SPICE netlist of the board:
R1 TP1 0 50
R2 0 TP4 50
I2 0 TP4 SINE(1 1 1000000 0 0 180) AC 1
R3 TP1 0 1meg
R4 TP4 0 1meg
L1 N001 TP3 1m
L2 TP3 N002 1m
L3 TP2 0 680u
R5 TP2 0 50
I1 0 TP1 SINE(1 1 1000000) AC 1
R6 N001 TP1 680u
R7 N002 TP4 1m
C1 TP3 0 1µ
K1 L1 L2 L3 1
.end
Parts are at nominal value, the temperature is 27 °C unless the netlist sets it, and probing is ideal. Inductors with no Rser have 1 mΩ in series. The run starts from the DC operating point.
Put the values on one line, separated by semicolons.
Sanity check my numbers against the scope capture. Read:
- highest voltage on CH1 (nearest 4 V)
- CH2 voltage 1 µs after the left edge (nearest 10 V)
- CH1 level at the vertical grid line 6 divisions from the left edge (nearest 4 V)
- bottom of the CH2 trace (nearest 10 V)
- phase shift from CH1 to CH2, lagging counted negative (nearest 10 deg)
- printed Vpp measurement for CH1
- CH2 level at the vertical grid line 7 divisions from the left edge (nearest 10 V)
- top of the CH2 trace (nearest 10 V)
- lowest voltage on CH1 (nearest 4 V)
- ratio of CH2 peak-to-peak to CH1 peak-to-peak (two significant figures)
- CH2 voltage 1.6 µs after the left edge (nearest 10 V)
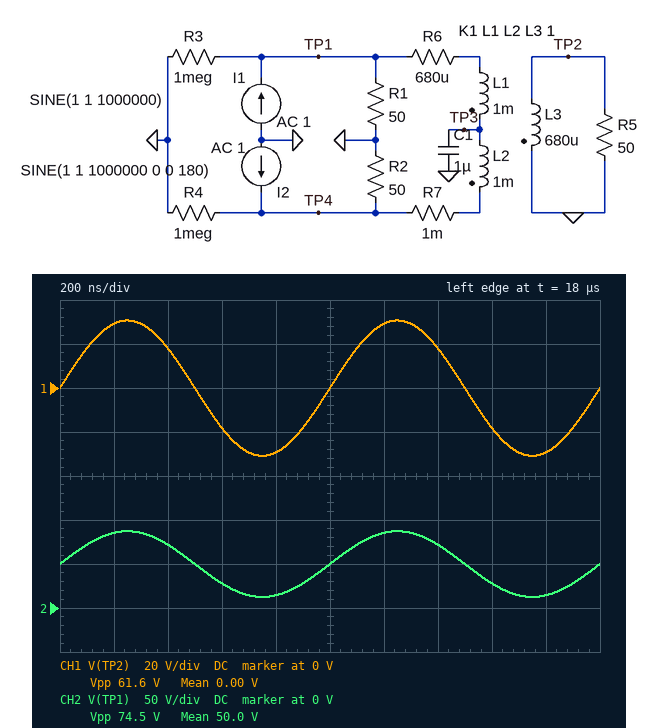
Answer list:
32 V; 50 V; 28 V; 10 V; 0 deg; 61.6 V; 70 V; 90 V; -32 V; 1.2; 30 V
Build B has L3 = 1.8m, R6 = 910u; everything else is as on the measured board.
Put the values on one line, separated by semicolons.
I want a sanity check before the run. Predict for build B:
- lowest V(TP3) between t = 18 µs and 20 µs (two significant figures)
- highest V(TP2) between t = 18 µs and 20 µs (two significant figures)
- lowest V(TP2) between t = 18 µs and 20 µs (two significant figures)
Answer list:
50 V; 35 V; -35 V
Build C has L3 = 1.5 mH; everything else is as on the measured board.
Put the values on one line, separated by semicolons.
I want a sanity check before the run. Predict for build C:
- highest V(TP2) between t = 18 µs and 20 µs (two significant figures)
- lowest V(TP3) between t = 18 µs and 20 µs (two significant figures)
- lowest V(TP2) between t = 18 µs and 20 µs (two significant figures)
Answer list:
35 V; 50 V; -35 V
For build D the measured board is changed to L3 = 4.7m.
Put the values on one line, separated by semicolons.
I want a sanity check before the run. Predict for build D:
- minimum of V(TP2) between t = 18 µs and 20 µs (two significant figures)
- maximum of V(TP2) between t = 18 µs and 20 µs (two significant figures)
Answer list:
-32 V; 32 V
